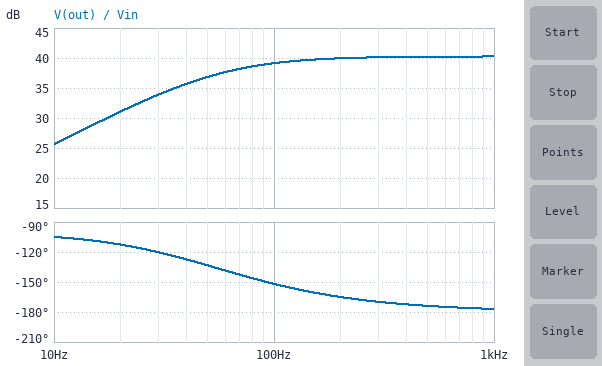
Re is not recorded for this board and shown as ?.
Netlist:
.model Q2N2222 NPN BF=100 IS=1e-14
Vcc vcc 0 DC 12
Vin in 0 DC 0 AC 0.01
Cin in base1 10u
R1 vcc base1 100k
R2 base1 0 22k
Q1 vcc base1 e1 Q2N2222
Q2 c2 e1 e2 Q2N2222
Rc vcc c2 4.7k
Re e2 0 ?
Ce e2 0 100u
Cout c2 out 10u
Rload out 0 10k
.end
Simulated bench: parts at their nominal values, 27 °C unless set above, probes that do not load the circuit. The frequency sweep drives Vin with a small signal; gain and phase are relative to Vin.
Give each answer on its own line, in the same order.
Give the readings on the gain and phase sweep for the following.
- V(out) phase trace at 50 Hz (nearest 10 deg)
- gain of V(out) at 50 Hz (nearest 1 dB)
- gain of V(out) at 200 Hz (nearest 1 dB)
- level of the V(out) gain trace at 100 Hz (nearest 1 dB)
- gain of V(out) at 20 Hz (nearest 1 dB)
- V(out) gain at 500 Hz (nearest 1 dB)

-130 deg
37 dB
40 dB
39 dB
31 dB
40 dB
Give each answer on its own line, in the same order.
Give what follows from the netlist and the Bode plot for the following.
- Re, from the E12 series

560 Ω
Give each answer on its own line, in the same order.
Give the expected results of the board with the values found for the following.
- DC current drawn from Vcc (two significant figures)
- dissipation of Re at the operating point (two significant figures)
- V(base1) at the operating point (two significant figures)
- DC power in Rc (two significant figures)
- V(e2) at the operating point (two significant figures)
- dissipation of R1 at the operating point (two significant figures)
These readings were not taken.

1.8 mA
1.6 mW
2.2 V
13 mW
940 mV
970 µW
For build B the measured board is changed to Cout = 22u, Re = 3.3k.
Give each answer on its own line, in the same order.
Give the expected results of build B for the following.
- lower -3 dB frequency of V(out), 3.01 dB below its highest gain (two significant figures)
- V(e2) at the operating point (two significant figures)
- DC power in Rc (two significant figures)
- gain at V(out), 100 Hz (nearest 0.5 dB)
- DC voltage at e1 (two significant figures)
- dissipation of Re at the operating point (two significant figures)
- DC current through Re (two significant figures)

10 Hz
1.0 V
450 µW
25.5 dB
1.7 V
320 µW
310 µA
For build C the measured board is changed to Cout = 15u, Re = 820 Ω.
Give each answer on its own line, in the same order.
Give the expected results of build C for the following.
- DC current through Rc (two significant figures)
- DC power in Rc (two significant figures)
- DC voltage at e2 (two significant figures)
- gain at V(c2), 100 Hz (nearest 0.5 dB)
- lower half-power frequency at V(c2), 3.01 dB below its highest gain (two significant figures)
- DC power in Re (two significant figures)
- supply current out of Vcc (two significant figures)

1.2 mA
6.4 mW
960 mV
36.5 dB
38 Hz
1.1 mW
1.3 mA
